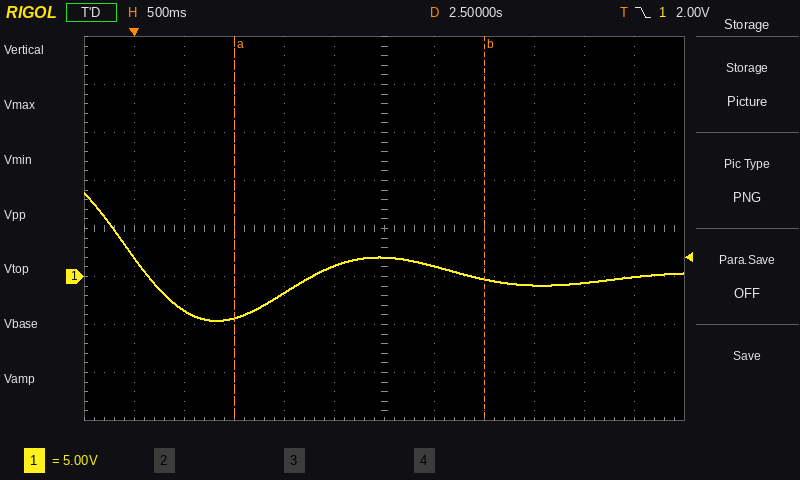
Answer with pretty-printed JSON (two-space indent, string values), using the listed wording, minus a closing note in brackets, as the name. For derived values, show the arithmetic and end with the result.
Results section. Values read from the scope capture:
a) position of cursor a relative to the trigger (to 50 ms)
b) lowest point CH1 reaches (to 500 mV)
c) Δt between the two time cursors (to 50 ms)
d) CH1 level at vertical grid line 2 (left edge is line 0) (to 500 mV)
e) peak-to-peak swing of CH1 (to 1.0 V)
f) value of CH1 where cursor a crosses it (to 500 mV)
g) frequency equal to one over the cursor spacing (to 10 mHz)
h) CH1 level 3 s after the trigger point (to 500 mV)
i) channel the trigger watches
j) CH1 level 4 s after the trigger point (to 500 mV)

{
  "position of cursor a relative to the trigger": "+1.00 s",
  "lowest point CH1 reaches": "-4.5 V",
  "Δt between the two time cursors": "2.50 s",
  "CH1 level at vertical grid line 2 (left edge is line 0)": "-3.5 V",
  "peak-to-peak swing of CH1": "13.0 V",
  "value of CH1 where cursor a crosses it": "-4.5 V",
  "frequency equal to one over the cursor spacing": "1 / 2.50 s ≈ 400 mHz",
  "CH1 level 3 s after the trigger point": "1.0 V",
  "channel the trigger watches": "CH1",
  "CH1 level 4 s after the trigger point": "-1.0 V"
}
